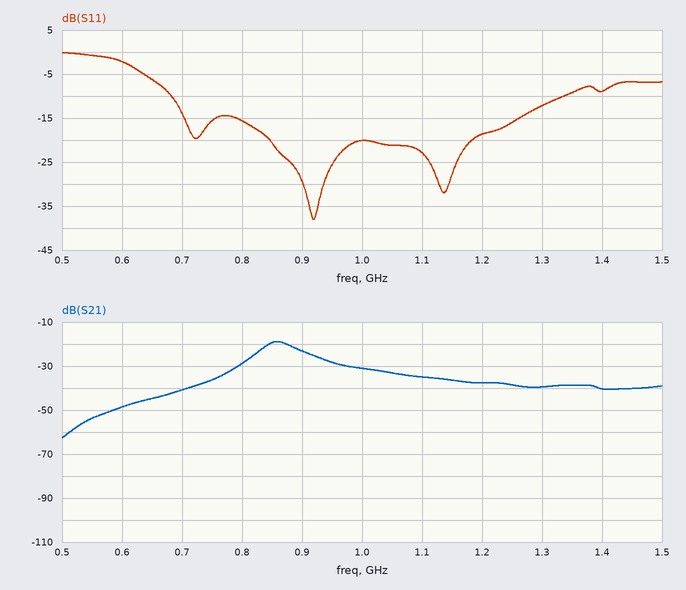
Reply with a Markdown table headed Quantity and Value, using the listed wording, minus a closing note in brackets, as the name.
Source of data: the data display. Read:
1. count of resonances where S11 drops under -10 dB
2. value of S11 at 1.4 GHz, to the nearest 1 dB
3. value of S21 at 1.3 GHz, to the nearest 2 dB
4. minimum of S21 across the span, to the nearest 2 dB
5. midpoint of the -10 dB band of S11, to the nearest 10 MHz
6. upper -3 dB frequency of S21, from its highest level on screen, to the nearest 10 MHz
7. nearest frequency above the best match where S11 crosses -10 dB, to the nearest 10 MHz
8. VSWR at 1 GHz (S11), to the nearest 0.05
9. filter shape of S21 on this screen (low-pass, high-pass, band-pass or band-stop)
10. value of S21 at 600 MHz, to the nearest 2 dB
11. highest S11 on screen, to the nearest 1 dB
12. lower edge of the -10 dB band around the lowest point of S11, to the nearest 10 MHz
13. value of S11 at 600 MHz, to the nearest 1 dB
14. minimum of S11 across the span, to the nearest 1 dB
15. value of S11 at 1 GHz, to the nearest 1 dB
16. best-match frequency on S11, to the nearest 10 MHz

| Quantity | Value |
|---|---|
| count of resonances where S11 drops under -10 dB | 3 |
| value of S11 at 1.4 GHz, to the nearest 1 dB | -9 dB |
| value of S21 at 1.3 GHz, to the nearest 2 dB | -40 dB |
| minimum of S21 across the span, to the nearest 2 dB | -62 dB |
| midpoint of the -10 dB band of S11, to the nearest 10 MHz | 1.01 GHz |
| upper -3 dB frequency of S21, from its highest level on screen, to the nearest 10 MHz | 890 MHz |
| nearest frequency above the best match where S11 crosses -10 dB, to the nearest 10 MHz | 1.34 GHz |
| VSWR at 1 GHz (S11), to the nearest 0.05 | 1.20 |
| filter shape of S21 on this screen | band-pass |
| value of S21 at 600 MHz, to the nearest 2 dB | -48 dB |
| highest S11 on screen, to the nearest 1 dB | 0 dB |
| lower edge of the -10 dB band around the lowest point of S11, to the nearest 10 MHz | 680 MHz |
| value of S11 at 600 MHz, to the nearest 1 dB | -2 dB |
| minimum of S11 across the span, to the nearest 1 dB | -38 dB |
| value of S11 at 1 GHz, to the nearest 1 dB | -20 dB |
| best-match frequency on S11, to the nearest 10 MHz | 920 MHz |
